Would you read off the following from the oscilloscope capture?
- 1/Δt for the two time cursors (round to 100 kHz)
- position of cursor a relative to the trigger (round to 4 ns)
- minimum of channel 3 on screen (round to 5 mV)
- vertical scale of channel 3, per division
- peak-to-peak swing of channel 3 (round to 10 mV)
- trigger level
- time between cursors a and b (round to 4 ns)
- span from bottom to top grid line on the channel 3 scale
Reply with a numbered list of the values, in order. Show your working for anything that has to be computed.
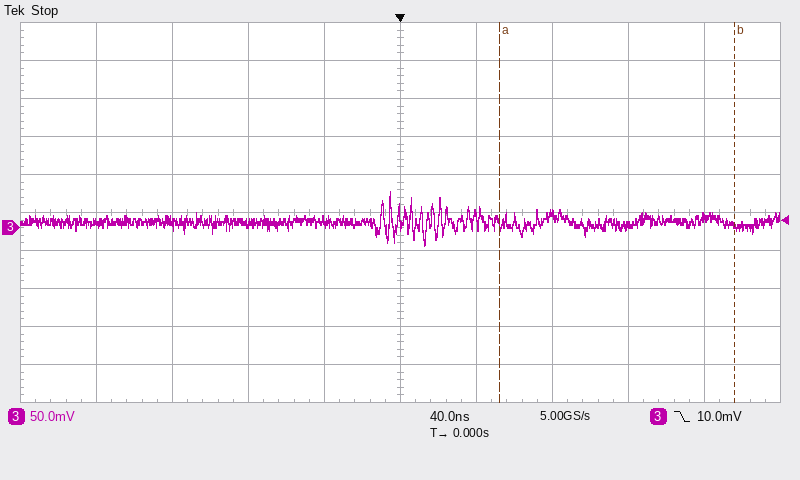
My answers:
1. 1 / 124 ns ≈ 8.1 MHz
2. +52 ns
3. -25 mV
4. 50 mV
5. 70 mV
6. 10.0 mV
7. 124 ns
8. 500 mV
